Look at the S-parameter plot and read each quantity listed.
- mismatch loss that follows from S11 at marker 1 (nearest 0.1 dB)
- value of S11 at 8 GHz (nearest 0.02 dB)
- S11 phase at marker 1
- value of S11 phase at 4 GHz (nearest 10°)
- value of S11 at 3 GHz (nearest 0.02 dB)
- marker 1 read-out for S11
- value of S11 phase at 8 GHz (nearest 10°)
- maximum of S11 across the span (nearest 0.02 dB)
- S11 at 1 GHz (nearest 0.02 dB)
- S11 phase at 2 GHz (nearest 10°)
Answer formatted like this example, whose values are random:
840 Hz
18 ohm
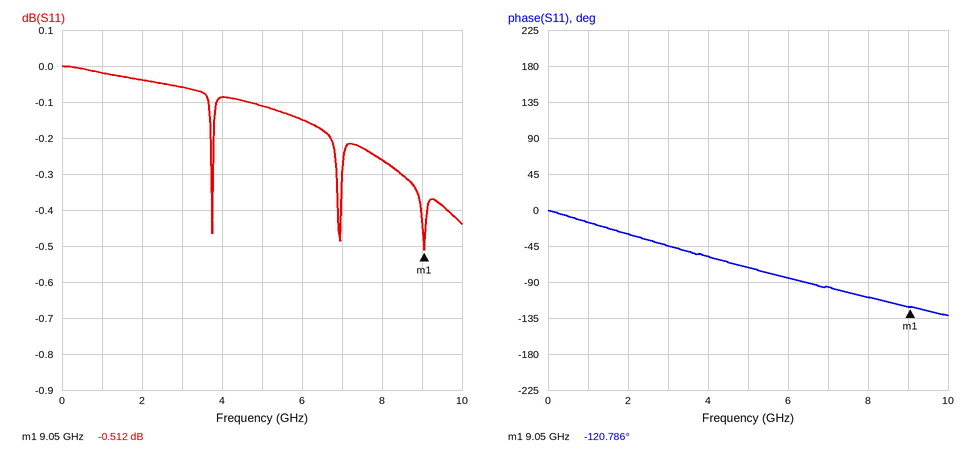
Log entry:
9.5 dB
-0.26 dB
-120.786°
-60°
-0.06 dB
-0.512 dB
-110°
0.00 dB
-0.02 dB
-30°
